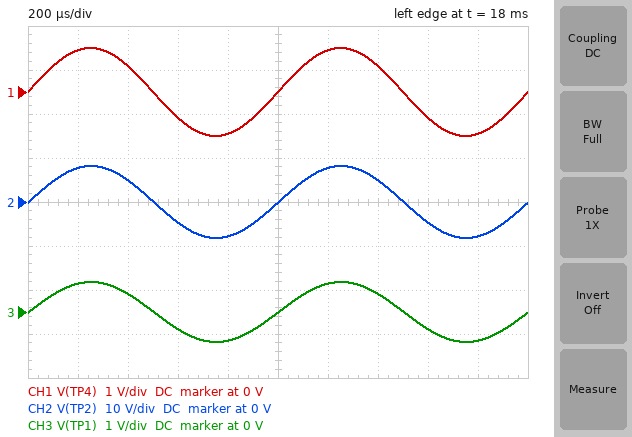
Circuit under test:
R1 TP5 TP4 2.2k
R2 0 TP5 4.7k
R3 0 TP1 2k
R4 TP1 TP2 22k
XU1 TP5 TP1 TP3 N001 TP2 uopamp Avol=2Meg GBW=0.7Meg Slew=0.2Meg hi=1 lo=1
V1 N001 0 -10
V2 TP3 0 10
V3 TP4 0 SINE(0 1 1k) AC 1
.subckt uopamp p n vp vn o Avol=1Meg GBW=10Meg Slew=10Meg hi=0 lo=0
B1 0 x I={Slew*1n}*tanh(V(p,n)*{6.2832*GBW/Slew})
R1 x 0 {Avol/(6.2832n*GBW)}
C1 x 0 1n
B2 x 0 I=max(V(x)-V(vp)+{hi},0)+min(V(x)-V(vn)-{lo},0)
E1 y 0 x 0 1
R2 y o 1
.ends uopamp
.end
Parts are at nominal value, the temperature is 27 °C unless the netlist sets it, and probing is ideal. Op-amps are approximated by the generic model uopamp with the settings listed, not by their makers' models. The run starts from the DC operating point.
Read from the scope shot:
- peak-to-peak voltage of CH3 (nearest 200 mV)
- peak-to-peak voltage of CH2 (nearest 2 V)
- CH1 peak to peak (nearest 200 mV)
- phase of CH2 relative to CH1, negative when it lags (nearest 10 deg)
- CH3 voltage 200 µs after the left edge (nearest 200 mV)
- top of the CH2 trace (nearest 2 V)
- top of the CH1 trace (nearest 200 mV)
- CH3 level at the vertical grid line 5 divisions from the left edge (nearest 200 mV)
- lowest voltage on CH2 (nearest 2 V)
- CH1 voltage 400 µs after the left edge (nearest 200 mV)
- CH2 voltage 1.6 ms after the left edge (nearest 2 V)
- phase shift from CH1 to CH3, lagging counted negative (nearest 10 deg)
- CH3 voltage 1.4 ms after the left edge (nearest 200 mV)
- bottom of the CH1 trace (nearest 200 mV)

1.4 V
16 V
2.0 V
0 deg
600 mV
8 V
1.0 V
0 V
-8 V
600 mV
-4 V
0 deg
400 mV
-1.0 V
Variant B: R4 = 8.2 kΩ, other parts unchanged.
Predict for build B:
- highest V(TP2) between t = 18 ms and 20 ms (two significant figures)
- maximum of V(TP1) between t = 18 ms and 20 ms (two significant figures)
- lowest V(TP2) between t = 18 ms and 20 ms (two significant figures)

3.5 V
680 mV
-3.5 V
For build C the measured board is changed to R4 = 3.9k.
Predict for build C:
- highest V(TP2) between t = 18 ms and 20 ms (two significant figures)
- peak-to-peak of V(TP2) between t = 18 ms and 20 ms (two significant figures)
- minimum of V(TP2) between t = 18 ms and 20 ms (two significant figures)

2.0 V
4.0 V
-2.0 V
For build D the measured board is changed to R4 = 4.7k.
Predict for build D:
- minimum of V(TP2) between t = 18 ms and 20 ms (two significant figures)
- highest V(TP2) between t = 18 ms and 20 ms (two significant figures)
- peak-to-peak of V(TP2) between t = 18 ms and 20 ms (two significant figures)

-2.3 V
2.3 V
4.6 V
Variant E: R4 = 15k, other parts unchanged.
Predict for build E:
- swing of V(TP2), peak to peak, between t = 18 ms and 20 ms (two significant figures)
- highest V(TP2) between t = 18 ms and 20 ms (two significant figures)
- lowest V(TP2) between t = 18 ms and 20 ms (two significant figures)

12 V
5.8 V
-5.8 V
